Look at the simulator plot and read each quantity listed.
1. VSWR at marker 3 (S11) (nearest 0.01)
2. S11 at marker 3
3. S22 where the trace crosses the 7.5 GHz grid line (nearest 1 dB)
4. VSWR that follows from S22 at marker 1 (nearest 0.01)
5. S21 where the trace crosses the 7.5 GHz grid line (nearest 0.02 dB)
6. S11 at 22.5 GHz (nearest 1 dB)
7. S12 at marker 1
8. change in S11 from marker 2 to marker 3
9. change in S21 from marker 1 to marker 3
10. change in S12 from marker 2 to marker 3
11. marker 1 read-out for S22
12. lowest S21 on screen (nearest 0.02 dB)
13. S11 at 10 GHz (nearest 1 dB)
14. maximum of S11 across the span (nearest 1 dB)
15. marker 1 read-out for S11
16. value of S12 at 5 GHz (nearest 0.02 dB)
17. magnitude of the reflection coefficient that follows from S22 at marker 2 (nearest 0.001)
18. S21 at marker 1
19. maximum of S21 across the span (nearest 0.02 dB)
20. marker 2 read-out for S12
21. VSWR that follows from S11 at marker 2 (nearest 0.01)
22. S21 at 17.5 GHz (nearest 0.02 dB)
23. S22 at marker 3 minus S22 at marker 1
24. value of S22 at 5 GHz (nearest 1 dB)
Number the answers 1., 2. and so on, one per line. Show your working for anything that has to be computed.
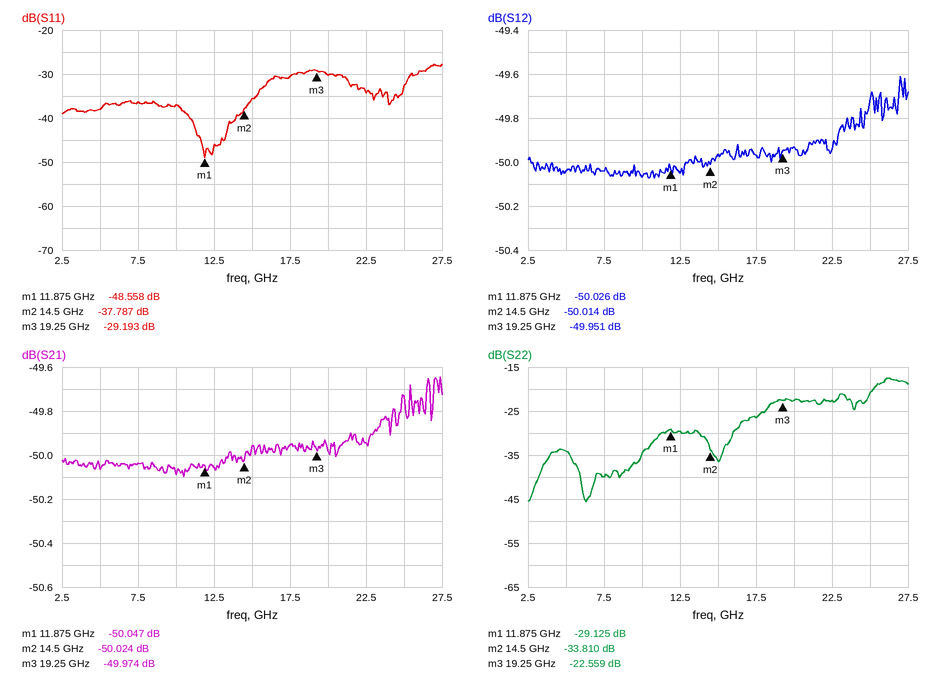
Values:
1. (1 + 0.0347)/(1 − 0.0347) ≈ 1.07
2. -29.193 dB
3. -40 dB
4. (1 + 0.0350)/(1 − 0.0350) ≈ 1.07
5. -50.04 dB
6. -34 dB
7. -50.026 dB
8. -29.193 − (-37.787) = 8.594 dB
9. -49.974 − (-50.047) = 0.073 dB
10. -49.951 − (-50.014) = 0.063 dB
11. -29.125 dB
12. -50.10 dB
13. -37 dB
14. -28 dB
15. -48.558 dB
16. -50.04 dB
17. 10^(-33.81/20) ≈ 0.020
18. -50.047 dB
19. -49.64 dB
20. -50.014 dB
21. (1 + 0.0129)/(1 − 0.0129) ≈ 1.03
22. -49.96 dB
23. -22.559 − (-29.125) = 6.566 dB
24. -34 dB
